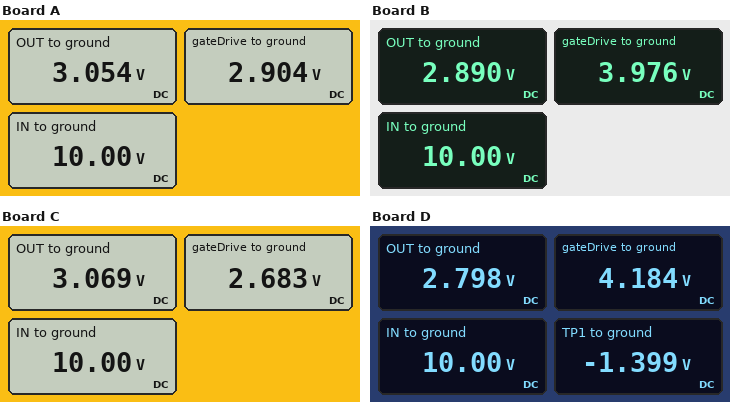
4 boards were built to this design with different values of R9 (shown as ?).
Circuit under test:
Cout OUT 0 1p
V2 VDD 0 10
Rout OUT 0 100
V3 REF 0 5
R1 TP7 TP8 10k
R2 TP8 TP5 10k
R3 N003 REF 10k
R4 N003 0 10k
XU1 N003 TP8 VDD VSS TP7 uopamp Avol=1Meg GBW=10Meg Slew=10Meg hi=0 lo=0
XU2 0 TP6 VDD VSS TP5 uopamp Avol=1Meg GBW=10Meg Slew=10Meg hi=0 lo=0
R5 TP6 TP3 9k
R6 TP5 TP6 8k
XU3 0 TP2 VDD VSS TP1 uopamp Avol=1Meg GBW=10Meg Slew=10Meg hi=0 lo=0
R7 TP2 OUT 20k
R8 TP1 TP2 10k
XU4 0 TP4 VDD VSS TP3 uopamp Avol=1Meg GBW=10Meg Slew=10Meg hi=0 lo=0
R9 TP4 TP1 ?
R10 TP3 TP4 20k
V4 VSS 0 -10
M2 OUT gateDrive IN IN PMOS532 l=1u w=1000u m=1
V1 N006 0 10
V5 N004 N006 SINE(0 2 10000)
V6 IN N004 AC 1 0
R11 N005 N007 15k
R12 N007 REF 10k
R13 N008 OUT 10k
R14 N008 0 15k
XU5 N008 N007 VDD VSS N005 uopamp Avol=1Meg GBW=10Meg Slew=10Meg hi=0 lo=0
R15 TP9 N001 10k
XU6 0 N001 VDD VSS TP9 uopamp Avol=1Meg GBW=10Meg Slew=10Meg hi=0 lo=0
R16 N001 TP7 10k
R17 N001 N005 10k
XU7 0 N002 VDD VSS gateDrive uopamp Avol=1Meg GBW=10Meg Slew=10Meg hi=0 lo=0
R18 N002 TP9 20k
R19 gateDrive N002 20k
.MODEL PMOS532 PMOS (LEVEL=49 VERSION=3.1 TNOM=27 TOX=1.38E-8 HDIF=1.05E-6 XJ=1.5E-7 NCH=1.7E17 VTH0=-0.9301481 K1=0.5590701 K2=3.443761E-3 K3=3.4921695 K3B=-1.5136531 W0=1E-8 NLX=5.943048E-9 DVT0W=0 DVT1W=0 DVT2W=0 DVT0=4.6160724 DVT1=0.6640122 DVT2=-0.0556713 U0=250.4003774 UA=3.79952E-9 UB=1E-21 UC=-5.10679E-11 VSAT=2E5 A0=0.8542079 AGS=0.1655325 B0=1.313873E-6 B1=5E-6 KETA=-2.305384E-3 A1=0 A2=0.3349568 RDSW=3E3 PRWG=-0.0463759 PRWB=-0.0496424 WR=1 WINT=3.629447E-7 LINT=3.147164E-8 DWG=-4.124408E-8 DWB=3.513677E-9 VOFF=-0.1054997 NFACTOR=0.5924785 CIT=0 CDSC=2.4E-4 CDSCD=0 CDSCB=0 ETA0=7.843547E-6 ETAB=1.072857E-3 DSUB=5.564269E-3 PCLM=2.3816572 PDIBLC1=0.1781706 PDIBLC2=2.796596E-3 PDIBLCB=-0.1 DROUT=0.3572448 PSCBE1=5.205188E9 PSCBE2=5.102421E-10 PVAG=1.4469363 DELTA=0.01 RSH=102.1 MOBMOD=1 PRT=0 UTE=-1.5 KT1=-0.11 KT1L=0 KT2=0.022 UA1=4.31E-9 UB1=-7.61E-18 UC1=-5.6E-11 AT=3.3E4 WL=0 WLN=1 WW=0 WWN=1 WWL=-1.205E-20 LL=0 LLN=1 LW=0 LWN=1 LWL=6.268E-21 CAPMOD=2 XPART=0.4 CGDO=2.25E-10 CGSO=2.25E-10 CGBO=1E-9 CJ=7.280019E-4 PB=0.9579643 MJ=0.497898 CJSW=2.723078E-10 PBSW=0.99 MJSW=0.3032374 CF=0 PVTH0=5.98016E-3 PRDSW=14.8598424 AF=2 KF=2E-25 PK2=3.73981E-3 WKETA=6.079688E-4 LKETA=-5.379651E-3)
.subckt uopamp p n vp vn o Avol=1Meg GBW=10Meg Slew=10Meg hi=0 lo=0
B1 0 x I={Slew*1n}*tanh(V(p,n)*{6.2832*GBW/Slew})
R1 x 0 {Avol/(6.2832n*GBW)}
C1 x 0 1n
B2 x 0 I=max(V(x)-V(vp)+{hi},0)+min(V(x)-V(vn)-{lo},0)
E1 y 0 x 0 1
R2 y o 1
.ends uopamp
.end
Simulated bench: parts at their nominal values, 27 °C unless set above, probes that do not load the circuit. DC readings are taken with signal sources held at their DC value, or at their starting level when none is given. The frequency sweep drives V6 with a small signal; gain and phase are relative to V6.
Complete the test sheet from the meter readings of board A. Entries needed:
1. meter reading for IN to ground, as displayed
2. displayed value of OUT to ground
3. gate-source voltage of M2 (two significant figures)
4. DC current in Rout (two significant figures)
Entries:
10.00 V
3.054 V
-7.1 V
31 mA
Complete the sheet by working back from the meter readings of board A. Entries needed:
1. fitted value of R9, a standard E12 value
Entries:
33 kΩ
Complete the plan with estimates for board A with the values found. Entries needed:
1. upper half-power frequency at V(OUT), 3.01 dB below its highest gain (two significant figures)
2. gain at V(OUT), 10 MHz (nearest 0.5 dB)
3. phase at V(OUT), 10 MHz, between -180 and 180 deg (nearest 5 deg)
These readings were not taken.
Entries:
660 MHz
-9.0 dB
0 deg
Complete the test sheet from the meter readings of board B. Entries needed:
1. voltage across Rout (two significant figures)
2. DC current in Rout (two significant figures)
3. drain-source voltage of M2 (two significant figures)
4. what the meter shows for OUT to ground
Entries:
2.9 V
29 mA
-7.1 V
2.890 V
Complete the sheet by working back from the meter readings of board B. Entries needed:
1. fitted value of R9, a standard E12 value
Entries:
12 kΩ
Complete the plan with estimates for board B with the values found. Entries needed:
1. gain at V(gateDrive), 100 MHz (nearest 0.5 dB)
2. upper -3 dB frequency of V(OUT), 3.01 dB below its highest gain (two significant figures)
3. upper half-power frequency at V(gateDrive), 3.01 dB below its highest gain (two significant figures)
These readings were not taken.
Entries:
-61.0 dB
460 MHz
3.1 MHz
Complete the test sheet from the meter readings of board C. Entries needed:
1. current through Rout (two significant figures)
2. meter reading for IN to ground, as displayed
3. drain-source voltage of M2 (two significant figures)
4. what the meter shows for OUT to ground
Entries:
31 mA
10.00 V
-6.9 V
3.069 V
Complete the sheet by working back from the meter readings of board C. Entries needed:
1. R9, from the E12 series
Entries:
47 kΩ
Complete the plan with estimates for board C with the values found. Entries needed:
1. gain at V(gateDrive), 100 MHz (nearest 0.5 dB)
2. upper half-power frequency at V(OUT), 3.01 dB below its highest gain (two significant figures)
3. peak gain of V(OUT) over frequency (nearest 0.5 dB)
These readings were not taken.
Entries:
-58.5 dB
690 MHz
-9.0 dB
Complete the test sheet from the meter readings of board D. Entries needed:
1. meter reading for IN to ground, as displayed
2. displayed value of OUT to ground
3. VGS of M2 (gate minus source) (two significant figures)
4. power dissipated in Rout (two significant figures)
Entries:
10.00 V
2.798 V
-5.8 V
78 mW
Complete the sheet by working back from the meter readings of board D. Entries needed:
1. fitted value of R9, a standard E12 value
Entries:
10 kΩ
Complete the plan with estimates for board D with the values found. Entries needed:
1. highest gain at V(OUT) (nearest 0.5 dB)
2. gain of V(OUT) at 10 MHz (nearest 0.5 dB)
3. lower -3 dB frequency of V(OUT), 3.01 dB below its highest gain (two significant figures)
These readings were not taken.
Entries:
-2.5 dB
-4.5 dB
2.1 MHz
